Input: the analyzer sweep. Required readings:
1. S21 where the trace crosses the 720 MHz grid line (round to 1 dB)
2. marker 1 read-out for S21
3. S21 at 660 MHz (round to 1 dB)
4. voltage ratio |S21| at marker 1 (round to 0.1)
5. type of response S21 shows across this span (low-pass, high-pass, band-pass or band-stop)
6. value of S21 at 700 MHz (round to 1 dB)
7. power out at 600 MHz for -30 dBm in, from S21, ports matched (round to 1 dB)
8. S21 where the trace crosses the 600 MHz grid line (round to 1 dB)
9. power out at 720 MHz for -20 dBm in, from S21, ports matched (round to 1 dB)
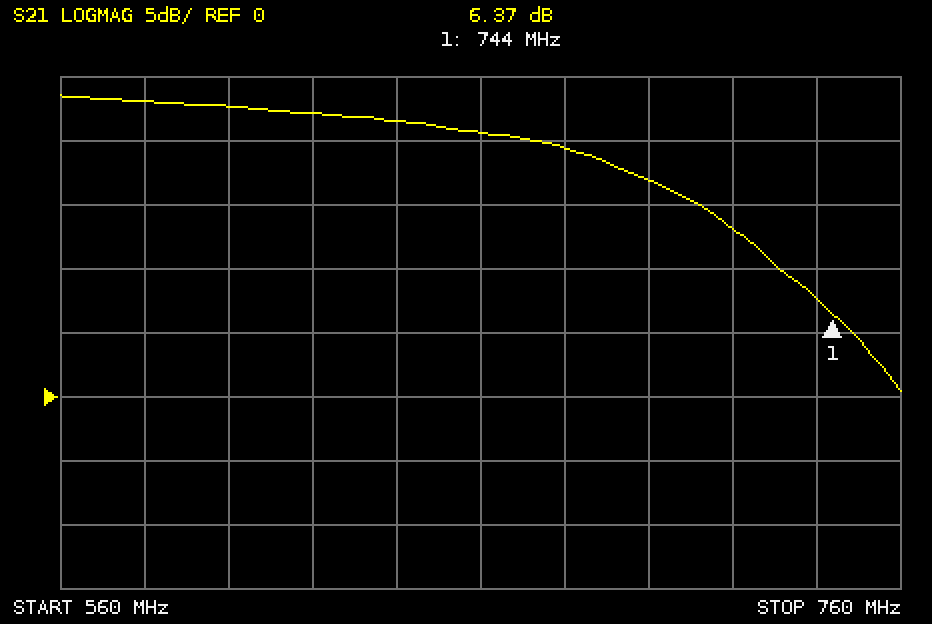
13 dB
6.37 dB
21 dB
2.1
low-pass
17 dB
-7 dBm
23 dB
-7 dBm
